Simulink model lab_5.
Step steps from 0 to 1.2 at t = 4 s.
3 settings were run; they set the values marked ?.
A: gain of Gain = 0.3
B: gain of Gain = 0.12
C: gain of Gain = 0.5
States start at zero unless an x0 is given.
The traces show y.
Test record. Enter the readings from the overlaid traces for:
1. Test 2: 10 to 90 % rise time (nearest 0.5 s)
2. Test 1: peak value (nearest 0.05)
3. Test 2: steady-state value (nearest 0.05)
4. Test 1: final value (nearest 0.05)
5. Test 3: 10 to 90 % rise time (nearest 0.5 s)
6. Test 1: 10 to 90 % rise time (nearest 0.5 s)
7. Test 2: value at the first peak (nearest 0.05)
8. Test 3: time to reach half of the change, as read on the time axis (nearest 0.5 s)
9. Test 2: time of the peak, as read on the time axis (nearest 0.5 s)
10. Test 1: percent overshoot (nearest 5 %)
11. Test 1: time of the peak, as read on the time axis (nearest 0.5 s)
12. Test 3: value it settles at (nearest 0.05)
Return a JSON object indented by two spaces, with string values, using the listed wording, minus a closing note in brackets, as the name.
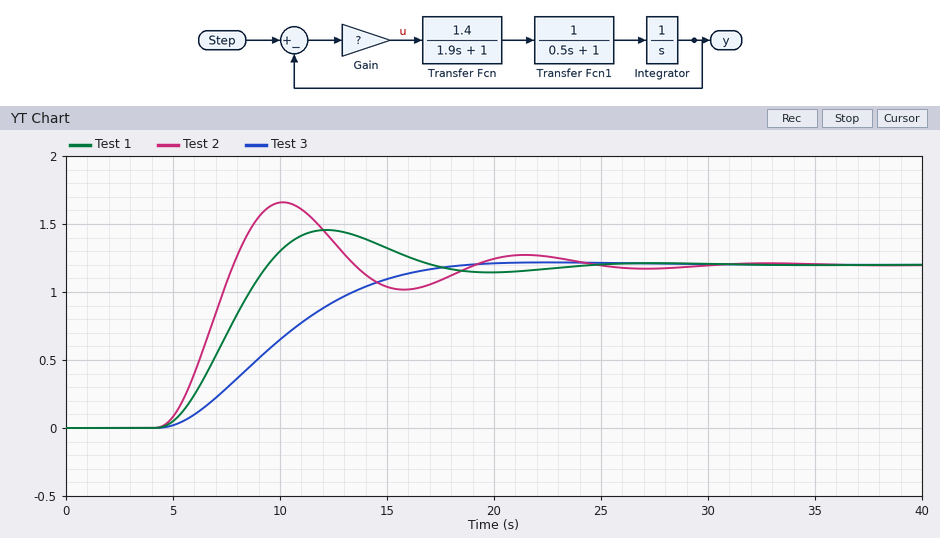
{
  "Test 2: 10 to 90 % rise time": "2.5 s",
  "Test 1: peak value": "1.45",
  "Test 2: steady-state value": "1.20",
  "Test 1: final value": "1.20",
  "Test 3: 10 to 90 % rise time": "8.5 s",
  "Test 1: 10 to 90 % rise time": "3.5 s",
  "Test 2: value at the first peak": "1.65",
  "Test 3: time to reach half of the change, as read on the time axis": "9.5 s",
  "Test 2: time of the peak, as read on the time axis": "10.0 s",
  "Test 1: percent overshoot": "20 %",
  "Test 1: time of the peak, as read on the time axis": "12.0 s",
  "Test 3: value it settles at": "1.20"
}
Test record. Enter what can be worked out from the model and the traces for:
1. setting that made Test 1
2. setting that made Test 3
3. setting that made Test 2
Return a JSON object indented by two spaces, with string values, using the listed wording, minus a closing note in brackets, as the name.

{
  "setting that made Test 1": "A",
  "setting that made Test 3": "B",
  "setting that made Test 2": "C"
}
